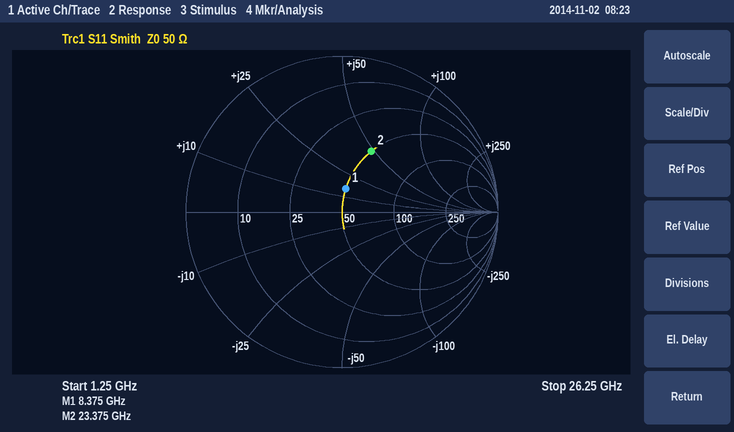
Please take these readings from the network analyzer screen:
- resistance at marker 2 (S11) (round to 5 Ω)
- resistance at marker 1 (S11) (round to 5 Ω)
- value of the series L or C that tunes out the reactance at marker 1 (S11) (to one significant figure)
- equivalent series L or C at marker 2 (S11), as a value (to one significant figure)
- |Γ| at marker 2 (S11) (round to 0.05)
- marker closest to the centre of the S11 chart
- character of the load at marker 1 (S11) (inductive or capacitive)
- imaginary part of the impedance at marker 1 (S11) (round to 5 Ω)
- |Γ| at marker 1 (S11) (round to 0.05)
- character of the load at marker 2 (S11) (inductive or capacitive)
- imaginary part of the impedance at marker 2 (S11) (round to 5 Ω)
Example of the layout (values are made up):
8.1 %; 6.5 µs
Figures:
50 Ω; 50 Ω; 1 pF; 300 pH; 0.45; marker 1; inductive; +15 Ω; 0.15; inductive; +50 Ω
